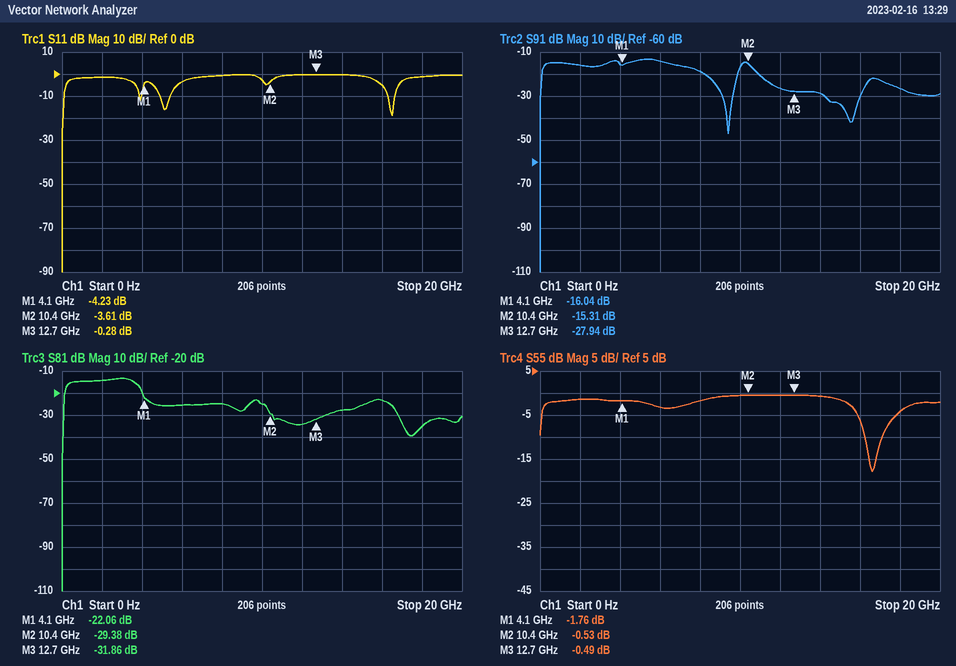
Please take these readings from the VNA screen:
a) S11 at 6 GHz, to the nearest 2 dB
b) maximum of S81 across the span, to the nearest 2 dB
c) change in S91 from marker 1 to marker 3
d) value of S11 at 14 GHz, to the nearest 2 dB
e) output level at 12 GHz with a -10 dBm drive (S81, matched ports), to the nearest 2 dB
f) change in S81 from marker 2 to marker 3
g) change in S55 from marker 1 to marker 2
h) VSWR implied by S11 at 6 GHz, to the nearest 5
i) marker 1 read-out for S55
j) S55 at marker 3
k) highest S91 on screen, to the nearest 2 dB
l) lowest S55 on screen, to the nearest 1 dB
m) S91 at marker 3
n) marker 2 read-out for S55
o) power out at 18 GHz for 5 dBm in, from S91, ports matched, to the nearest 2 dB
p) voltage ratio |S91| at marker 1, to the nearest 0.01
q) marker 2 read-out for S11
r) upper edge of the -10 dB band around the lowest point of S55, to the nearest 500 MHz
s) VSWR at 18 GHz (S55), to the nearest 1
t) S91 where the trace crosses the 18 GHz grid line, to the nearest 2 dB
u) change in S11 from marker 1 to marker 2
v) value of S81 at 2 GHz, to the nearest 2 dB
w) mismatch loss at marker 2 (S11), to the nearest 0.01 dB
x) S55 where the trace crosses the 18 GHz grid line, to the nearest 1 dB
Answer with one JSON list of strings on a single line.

["-4 dB", "-14 dB", "-11.90 dB", "0 dB", "-44 dBm", "-2.48 dB", "1.23 dB", "5", "-1.76 dB", "-0.49 dB", "-14 dB", "-18 dB", "-27.94 dB", "-0.53 dB", "-22 dBm", "0.16", "-3.61 dB", "17.0 GHz", "4", "-26 dB", "0.62 dB", "-14 dB", "2.48 dB", "-4 dB"]
